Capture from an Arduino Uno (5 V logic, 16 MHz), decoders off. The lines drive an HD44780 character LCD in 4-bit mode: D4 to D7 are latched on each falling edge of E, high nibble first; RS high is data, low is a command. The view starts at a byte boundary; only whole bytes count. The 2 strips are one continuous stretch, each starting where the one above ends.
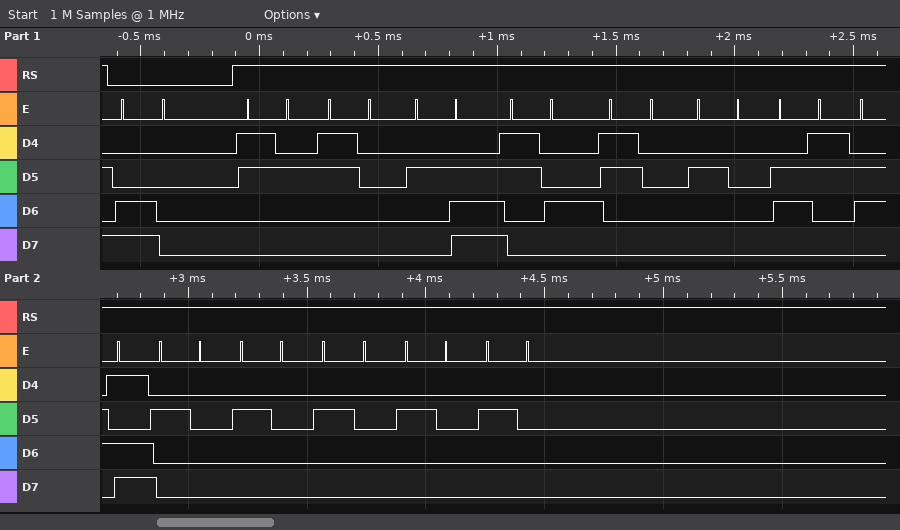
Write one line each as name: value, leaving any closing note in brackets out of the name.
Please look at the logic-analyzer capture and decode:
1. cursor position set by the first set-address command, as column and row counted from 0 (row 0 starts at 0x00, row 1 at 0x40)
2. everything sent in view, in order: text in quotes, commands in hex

cursor position set by the first set-address command, as column and row counted from 0: column 0, row 1
everything sent in view, in order: text in quotes, commands in hex: 0xC0 "20.40 cm     "
